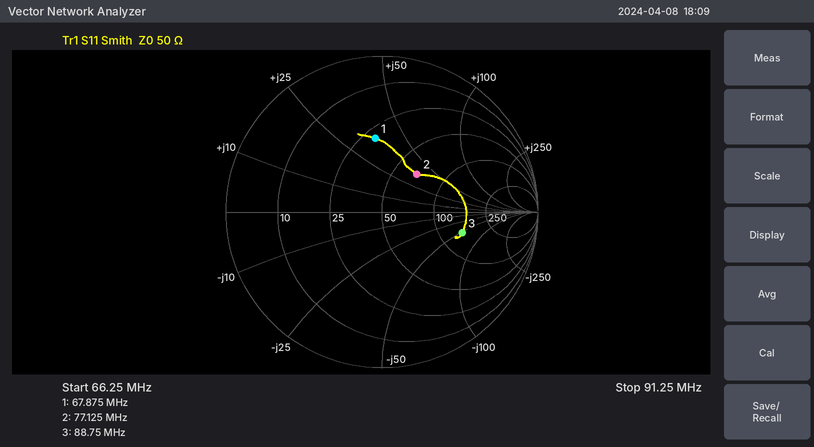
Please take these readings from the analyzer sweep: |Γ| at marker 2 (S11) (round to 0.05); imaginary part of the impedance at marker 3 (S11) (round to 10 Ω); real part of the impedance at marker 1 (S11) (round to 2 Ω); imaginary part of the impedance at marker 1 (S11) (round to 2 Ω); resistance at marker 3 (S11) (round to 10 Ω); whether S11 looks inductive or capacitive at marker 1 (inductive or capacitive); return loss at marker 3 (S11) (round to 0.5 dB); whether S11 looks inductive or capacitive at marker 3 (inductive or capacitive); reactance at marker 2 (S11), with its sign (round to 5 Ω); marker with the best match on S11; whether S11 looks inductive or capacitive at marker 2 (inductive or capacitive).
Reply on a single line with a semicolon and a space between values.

0.35; -50 Ω; 30 Ω; +36 Ω; 140 Ω; inductive; 5.5 dB; capacitive; +35 Ω; marker 2; inductive
